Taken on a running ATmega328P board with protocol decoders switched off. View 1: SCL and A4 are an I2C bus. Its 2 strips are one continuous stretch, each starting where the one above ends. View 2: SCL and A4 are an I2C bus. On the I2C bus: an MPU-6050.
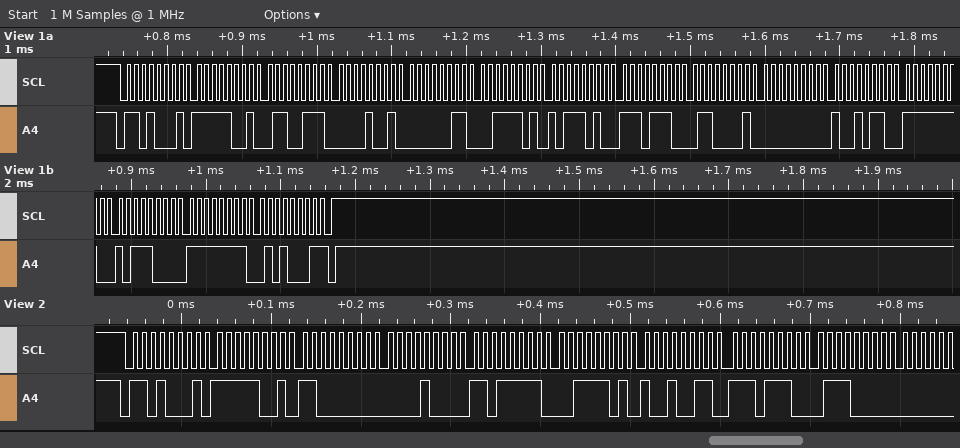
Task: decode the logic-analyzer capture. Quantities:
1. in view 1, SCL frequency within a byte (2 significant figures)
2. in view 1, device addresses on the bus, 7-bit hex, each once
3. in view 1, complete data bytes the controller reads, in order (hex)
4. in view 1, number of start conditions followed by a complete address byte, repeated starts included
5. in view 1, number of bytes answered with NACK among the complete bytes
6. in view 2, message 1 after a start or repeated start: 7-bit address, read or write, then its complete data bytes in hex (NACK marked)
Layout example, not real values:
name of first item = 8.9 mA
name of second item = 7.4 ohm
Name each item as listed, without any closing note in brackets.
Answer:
in view 1, SCL frequency within a byte = 100 kHz
in view 1, device addresses on the bus, 7-bit hex, each once = 0x68
in view 1, complete data bytes the controller reads, in order = F9 67 09 03 3D BA EE 61 00 96 FE B8 FF 51
in view 1, number of start conditions followed by a complete address byte, repeated starts included = 1
in view 1, number of bytes answered with NACK among the complete bytes = 1
in view 2, message 1 after a start or repeated start: 7-bit address, read or write, then its complete data bytes in hex = 0x68 read: F9 C0 08 DF 3D 93 EE 70
